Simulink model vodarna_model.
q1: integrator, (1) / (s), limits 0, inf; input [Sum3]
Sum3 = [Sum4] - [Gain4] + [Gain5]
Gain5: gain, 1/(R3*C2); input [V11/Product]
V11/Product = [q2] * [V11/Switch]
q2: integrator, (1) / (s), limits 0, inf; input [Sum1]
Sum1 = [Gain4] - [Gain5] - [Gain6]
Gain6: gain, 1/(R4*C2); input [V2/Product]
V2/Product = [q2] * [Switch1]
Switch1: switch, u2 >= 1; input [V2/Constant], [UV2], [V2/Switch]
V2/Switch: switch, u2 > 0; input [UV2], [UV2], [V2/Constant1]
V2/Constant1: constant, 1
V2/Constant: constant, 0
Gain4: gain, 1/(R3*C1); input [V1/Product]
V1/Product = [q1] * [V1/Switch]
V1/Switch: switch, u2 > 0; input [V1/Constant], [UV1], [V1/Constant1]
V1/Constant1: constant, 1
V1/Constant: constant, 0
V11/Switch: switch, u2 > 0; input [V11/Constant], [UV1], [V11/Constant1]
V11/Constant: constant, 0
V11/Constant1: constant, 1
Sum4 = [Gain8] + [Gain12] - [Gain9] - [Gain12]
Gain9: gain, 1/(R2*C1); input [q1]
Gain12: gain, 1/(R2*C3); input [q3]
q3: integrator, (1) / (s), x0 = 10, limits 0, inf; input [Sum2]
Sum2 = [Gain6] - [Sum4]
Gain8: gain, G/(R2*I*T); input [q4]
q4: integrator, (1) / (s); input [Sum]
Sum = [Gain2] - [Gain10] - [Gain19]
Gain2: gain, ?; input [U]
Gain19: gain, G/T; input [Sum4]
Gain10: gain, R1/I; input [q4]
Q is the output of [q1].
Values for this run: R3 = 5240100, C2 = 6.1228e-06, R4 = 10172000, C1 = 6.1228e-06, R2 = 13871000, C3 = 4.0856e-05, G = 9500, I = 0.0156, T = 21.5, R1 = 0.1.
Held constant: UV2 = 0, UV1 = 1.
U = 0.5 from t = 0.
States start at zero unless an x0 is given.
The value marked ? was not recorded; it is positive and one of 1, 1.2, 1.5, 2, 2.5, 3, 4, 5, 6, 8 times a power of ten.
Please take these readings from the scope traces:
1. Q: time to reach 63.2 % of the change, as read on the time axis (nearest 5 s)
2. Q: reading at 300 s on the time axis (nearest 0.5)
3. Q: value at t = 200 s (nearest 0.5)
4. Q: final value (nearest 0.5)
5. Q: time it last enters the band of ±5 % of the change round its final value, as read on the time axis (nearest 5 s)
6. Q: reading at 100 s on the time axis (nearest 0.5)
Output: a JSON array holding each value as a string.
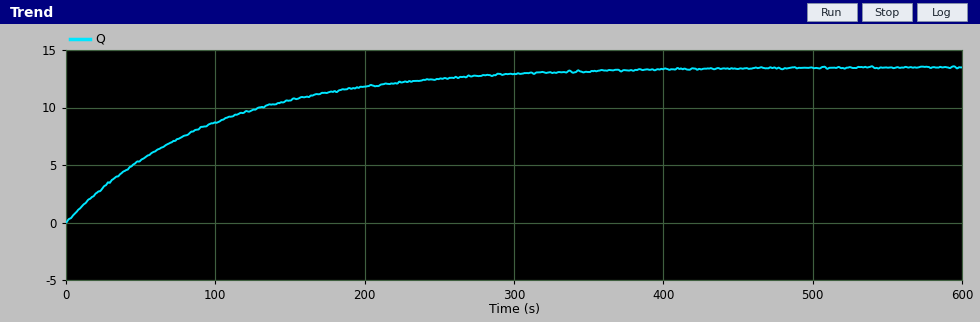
["95 s", "13.0", "12.0", "13.5", "290 s", "8.5"]
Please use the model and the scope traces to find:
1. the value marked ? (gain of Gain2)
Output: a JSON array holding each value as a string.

["1000"]
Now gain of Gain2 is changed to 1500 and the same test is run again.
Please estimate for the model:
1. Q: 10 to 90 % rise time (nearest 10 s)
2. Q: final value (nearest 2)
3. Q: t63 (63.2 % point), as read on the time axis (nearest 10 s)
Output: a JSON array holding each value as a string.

["210 s", "20", "100 s"]
